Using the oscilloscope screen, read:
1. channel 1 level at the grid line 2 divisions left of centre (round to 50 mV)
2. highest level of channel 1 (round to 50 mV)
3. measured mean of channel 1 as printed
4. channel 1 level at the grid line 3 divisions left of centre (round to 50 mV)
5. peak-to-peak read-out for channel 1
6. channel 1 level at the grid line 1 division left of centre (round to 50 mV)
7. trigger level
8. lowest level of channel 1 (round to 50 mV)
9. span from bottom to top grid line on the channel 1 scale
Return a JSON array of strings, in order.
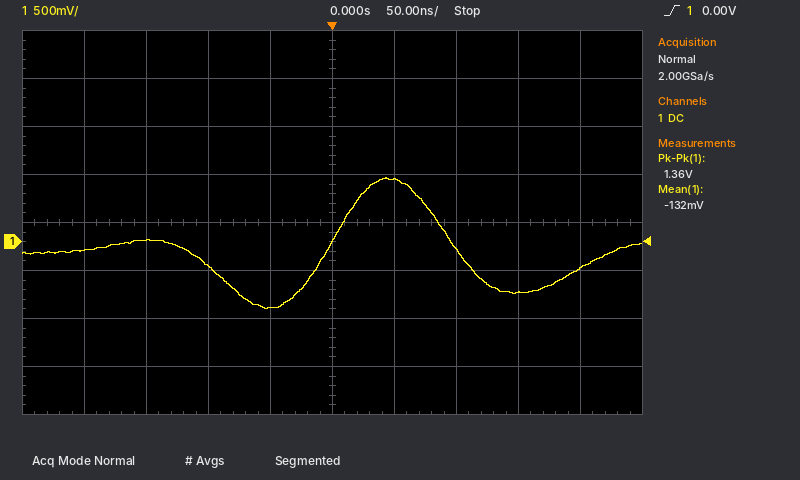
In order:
["-250 mV", "650 mV", "-132 mV", "0 mV", "1.36 V", "-700 mV", "0.00 V", "-700 mV", "4 V"]
